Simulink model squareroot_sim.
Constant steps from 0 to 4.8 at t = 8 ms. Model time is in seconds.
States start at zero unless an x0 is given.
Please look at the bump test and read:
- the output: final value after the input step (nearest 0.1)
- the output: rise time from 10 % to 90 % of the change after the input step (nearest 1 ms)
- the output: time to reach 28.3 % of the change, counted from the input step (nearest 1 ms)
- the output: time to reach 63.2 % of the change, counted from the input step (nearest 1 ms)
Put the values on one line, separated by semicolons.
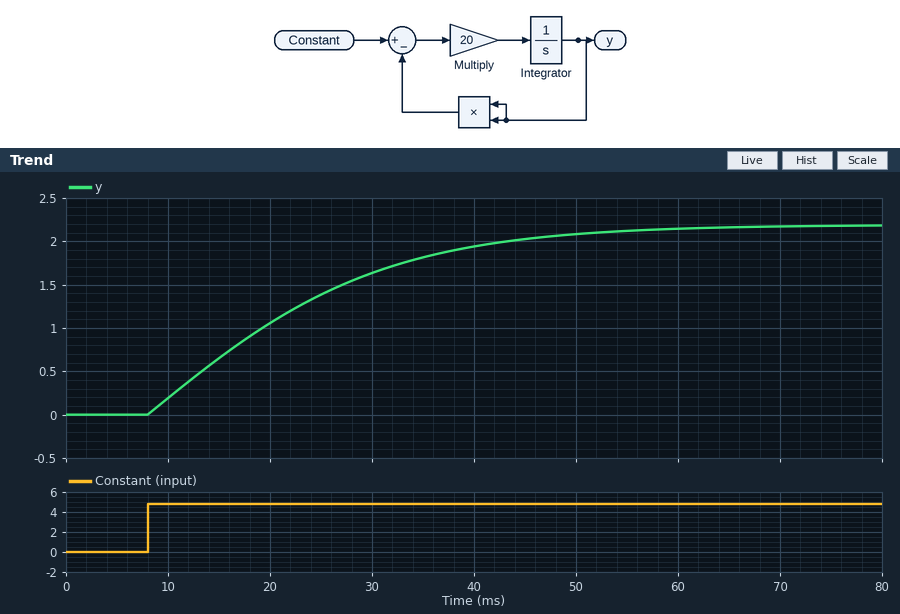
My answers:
2.2; 31 ms; 7 ms; 17 ms
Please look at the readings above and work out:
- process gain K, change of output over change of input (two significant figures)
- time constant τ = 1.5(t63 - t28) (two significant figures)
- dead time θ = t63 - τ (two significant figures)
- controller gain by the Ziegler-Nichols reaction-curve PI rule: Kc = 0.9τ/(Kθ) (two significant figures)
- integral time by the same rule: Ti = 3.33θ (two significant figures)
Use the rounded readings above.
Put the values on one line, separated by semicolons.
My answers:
0.46; 15 ms; 2.0 ms; 15; 6.7 ms
